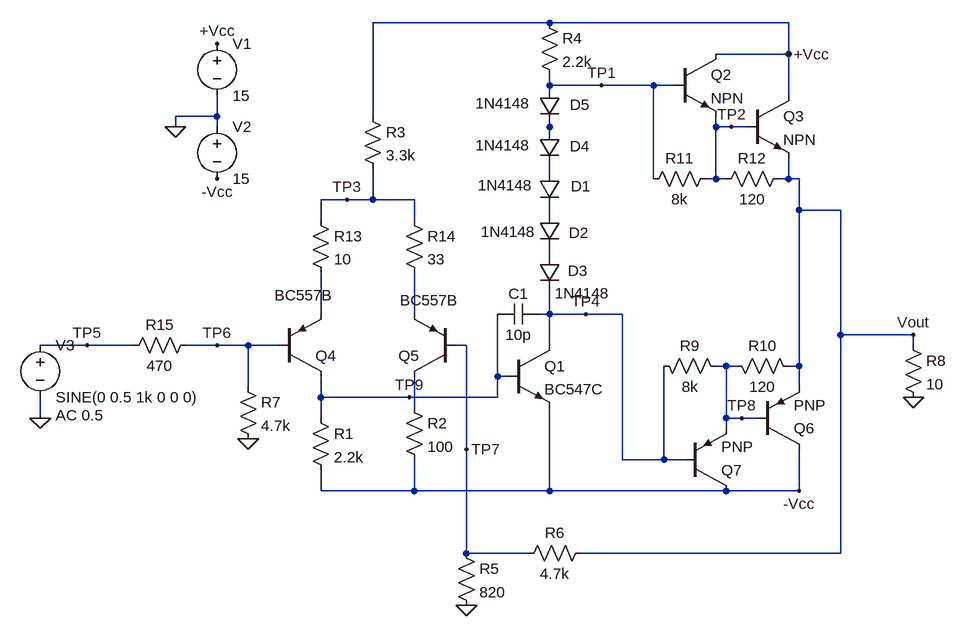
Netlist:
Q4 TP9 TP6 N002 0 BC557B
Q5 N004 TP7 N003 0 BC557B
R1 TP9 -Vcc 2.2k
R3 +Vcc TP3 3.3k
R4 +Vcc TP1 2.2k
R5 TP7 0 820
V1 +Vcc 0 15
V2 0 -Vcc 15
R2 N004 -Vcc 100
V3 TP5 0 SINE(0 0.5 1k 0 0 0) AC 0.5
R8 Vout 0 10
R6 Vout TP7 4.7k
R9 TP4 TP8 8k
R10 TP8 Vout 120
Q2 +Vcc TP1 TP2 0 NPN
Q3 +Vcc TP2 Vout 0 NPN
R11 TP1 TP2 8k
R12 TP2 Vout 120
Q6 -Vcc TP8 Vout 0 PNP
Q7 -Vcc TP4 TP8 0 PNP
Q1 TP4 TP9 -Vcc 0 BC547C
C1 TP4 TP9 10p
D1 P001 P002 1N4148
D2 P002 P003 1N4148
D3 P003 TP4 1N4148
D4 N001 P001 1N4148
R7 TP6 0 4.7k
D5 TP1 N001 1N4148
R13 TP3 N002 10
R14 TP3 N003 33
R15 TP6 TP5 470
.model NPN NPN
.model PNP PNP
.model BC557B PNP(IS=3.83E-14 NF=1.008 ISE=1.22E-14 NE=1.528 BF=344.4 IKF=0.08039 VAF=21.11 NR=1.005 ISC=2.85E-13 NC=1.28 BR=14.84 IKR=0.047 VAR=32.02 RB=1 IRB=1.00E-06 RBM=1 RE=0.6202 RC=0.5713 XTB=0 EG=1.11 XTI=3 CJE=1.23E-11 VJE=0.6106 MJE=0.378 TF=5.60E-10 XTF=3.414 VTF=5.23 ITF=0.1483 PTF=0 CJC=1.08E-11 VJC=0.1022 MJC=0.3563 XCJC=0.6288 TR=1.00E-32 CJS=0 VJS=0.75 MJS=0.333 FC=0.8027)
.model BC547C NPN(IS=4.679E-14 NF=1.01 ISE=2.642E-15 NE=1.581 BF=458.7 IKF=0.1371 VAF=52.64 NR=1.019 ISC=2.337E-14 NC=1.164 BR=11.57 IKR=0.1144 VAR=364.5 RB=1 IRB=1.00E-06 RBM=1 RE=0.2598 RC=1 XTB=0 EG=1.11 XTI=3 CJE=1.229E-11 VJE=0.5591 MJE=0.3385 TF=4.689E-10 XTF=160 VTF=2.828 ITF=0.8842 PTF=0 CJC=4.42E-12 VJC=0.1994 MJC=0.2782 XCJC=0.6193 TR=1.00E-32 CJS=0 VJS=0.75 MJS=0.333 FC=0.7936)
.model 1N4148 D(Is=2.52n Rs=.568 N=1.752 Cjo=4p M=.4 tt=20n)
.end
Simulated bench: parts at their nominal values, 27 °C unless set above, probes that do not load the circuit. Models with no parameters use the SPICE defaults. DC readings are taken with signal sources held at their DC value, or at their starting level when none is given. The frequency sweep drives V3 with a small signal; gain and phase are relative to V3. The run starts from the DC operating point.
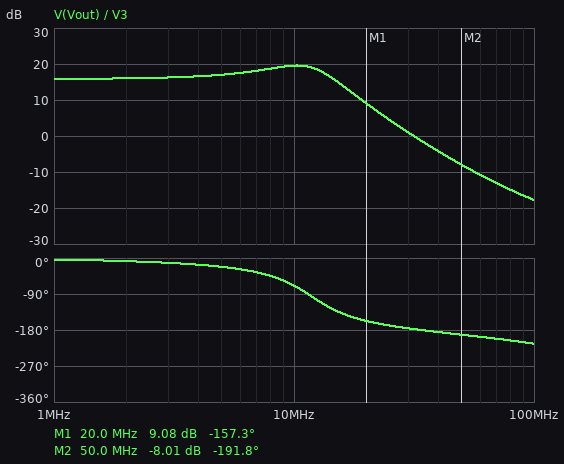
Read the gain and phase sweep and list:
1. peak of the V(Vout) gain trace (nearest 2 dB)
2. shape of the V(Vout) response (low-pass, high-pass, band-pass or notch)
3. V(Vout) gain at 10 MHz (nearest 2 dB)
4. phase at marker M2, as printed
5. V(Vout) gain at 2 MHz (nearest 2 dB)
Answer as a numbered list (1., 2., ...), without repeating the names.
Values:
1. 20 dB
2. low-pass
3. 20 dB
4. -191.8 deg
5. 16 dB
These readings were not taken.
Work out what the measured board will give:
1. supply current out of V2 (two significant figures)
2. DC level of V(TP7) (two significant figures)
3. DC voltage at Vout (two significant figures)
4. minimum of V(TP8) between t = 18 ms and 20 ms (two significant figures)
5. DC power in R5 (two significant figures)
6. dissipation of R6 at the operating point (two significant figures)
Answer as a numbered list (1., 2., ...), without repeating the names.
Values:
1. 160 mA
2. -200 mV
3. -1.4 V
4. -5.4 V
5. 49 µW
6. 300 µW
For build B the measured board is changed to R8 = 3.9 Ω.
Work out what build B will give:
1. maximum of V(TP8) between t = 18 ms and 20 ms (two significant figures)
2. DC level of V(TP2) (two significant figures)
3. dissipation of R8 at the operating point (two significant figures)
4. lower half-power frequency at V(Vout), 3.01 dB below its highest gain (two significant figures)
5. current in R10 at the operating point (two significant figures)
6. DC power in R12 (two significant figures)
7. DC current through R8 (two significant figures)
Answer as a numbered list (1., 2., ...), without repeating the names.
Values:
1. 1.0 V
2. -600 mV
3. 490 mW
4. 3.9 MHz
5. 7.7 mA
6. 5.1 mW
7. 350 mA
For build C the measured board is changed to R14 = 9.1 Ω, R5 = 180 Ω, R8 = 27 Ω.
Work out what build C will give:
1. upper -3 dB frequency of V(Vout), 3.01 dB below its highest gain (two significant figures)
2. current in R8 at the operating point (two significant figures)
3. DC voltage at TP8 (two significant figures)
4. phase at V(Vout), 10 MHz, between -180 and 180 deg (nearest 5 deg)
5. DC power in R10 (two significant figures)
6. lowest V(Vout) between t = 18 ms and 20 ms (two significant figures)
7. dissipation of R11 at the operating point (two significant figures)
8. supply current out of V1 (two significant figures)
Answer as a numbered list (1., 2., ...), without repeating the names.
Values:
1. 6.3 MHz
2. 100 mA
3. -3.7 V
4. -120 deg
5. 6.7 mW
6. -13 V
7. 85 µW
8. 30 mA
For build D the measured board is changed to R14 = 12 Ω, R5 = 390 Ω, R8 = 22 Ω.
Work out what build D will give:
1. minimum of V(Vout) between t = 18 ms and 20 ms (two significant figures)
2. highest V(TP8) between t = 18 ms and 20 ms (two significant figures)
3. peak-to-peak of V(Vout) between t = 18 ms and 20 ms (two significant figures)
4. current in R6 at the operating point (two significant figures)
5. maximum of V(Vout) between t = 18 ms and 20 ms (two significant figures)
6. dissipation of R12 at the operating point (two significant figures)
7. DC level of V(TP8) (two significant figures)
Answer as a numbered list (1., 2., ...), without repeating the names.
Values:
1. -7.5 V
2. 3.7 V
3. 12 V
4. 300 µA
5. 4.4 V
6. 5.7 mW
7. -2.4 V
